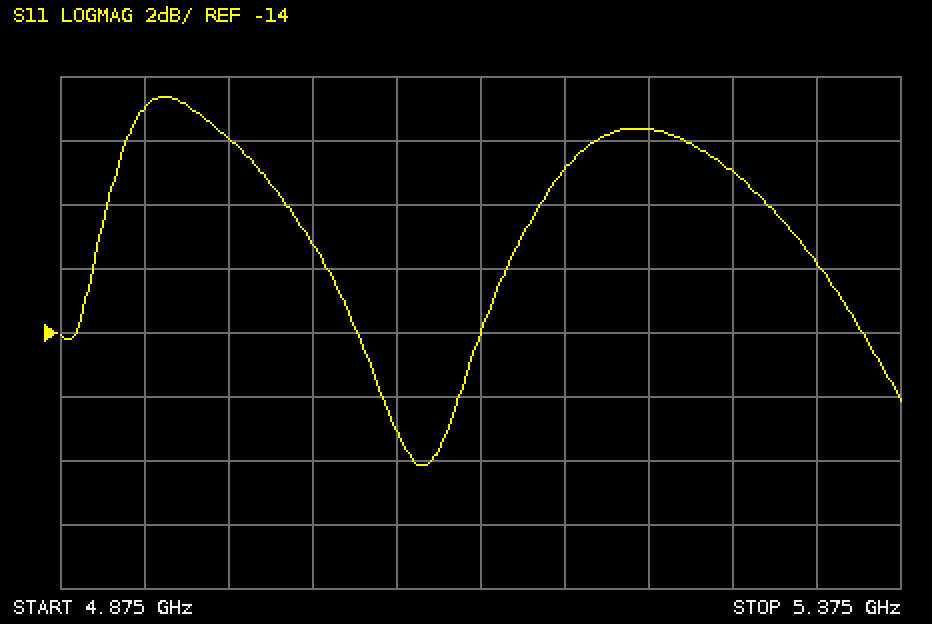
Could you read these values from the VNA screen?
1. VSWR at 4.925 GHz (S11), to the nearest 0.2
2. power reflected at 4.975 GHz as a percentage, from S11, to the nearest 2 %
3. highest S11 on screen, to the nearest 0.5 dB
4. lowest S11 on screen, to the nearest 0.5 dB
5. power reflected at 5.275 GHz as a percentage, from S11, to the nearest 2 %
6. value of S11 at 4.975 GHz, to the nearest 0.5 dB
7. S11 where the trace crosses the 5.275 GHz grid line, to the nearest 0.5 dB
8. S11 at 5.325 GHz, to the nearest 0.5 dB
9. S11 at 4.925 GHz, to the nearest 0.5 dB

2.6
16 %
-6.5 dB
-18.0 dB
12 %
-8.0 dB
-9.0 dB
-12.0 dB
-7.0 dB
